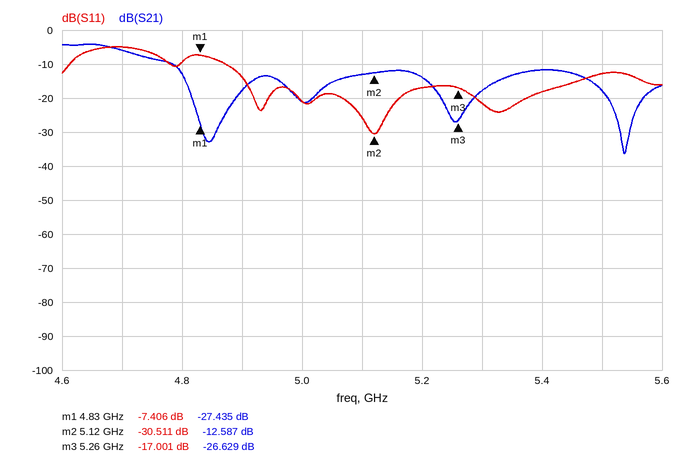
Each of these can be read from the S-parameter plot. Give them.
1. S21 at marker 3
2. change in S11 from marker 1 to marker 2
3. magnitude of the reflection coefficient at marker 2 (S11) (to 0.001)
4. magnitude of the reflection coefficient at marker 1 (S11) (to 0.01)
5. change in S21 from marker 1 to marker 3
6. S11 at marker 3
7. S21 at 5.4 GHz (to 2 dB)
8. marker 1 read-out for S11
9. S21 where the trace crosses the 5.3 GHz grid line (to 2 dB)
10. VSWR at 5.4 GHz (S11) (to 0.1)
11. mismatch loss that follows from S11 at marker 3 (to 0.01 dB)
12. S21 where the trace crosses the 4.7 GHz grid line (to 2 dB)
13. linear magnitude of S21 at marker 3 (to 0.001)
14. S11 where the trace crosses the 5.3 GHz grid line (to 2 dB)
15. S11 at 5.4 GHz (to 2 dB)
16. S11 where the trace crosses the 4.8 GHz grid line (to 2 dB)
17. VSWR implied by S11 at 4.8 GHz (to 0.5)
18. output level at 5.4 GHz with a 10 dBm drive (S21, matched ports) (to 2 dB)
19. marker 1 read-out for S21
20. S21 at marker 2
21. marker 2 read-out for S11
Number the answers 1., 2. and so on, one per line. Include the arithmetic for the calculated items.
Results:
1. -26.629 dB
2. -30.511 − (-7.406) = -23.105 dB
3. 10^(-30.511/20) ≈ 0.030
4. 10^(-7.406/20) ≈ 0.43
5. -26.629 − (-27.435) = 0.806 dB
6. -17.001 dB
7. -12 dB
8. -7.406 dB
9. -18 dB
10. |Γ| = 10^(-18/20) = 0.1259; VSWR = (1 + 0.1259)/(1 − 0.1259) ≈ 1.3
11. −10 log10(1 − 10^(-17.001/10)) ≈ 0.09 dB
12. -6 dB
13. 10^(-26.629/20) ≈ 0.047
14. -22 dB
15. -18 dB
16. -10 dB
17. |Γ| = 10^(-10/20) = 0.3162; VSWR = (1 + 0.3162)/(1 − 0.3162) ≈ 1.92, so 2.0 to the nearest 0.5
18. 10 dBm + (-12 dB) = -2 dBm
19. -27.435 dB
20. -12.587 dB
21. -30.511 dB
